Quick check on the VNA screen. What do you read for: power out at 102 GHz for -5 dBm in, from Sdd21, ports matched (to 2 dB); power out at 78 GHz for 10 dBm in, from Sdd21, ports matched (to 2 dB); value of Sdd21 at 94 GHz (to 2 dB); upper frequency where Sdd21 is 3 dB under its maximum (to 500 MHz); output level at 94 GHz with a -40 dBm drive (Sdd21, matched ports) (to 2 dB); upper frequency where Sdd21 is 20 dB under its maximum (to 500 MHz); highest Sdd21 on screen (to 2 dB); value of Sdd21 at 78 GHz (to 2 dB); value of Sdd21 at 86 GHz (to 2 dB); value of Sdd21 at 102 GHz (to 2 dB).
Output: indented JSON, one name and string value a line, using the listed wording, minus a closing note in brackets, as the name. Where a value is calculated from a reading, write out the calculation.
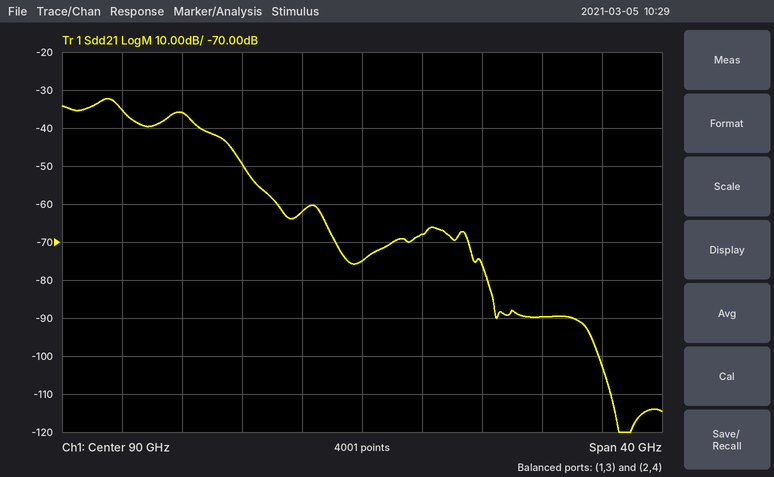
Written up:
{
  "power out at 102 GHz for -5 dBm in, from Sdd21, ports matched": "-5 dBm + (-90 dB) = -94 dBm",
  "power out at 78 GHz for 10 dBm in, from Sdd21, ports matched": "10 dBm + (-36 dB) = -26 dBm",
  "value of Sdd21 at 94 GHz": "-68 dB",
  "upper frequency where Sdd21 is 3 dB under its maximum": "74.0 GHz",
  "output level at 94 GHz with a -40 dBm drive (Sdd21, matched ports)": "-40 dBm + (-68 dB) = -108 dBm",
  "upper frequency where Sdd21 is 20 dB under its maximum": "82.5 GHz",
  "highest Sdd21 on screen": "-32 dB",
  "value of Sdd21 at 78 GHz": "-36 dB",
  "value of Sdd21 at 86 GHz": "-62 dB",
  "value of Sdd21 at 102 GHz": "-90 dB"
}
